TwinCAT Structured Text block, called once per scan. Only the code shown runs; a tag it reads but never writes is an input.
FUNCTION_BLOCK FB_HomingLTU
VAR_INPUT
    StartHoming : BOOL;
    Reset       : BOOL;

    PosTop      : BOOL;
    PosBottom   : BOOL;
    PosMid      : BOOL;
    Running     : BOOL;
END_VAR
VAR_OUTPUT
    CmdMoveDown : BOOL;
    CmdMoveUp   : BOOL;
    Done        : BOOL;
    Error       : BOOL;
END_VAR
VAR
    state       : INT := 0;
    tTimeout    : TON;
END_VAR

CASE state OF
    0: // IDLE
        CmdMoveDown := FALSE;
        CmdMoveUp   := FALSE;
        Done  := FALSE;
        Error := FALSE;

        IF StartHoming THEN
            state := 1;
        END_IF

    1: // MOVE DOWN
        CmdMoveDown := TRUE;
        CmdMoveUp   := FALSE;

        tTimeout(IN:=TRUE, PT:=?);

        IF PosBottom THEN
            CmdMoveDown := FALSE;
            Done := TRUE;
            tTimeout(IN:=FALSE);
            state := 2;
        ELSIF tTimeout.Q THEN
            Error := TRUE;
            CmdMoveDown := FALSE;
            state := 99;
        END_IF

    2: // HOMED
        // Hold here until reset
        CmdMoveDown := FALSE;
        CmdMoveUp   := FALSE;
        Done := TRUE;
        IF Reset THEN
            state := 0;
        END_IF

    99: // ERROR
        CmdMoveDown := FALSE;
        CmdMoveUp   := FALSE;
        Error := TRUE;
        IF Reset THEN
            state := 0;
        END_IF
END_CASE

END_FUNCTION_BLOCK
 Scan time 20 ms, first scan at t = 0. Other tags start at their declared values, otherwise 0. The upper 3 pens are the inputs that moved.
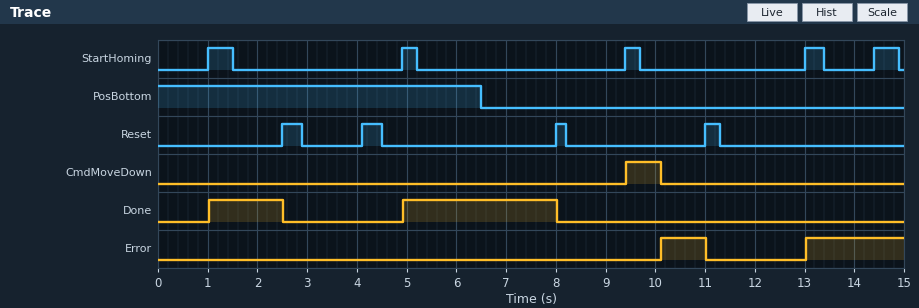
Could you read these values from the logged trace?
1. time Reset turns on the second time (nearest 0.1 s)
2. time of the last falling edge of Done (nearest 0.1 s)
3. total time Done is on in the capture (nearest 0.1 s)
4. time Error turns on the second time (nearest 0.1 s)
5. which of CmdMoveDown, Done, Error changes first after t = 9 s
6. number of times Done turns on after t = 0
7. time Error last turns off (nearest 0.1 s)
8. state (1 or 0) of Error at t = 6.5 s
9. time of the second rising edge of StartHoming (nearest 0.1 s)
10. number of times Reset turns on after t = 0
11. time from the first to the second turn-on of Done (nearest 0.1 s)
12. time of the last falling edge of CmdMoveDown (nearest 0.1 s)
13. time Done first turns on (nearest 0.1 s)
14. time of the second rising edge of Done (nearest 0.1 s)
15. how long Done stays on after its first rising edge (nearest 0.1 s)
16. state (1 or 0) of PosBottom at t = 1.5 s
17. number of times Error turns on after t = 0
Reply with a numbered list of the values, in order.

1. 4.1 s
2. 8.0 s
3. 4.6 s
4. 13.0 s
5. CmdMoveDown
6. 2
7. 11.0 s
8. 0
9. 4.9 s
10. 4
11. 3.9 s
12. 10.1 s
13. 1.0 s
14. 4.9 s
15. 1.5 s
16. 1
17. 2
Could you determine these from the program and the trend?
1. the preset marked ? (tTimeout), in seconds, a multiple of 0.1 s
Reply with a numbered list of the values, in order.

1. 0.7 s
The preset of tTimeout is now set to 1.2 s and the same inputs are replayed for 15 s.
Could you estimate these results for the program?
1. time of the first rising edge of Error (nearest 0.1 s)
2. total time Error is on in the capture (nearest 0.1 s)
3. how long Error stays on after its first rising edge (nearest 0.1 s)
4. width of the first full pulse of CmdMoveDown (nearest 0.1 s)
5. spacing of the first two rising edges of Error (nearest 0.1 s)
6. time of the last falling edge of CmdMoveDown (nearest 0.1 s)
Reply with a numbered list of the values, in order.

1. 10.6 s
2. 2.4 s
3. 0.4 s
4. 1.2 s
5. 2.4 s
6. 10.6 s
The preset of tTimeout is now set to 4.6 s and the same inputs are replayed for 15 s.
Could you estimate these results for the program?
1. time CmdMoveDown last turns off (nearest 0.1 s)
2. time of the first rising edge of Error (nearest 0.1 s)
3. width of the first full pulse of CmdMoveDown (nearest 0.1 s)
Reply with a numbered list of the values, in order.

1. 14.0 s
2. 14.0 s
3. 4.6 s
